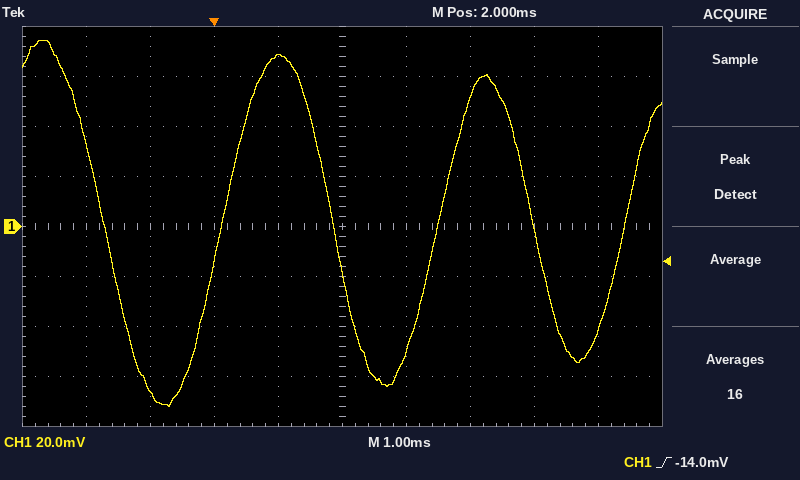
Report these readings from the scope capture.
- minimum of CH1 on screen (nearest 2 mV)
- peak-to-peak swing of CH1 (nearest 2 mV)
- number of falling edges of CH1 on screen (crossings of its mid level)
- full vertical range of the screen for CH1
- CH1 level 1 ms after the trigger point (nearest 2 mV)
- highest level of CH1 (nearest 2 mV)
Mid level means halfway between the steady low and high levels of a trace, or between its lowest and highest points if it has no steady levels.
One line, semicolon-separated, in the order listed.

-72 mV; 146 mV; 3; 160 mV; 68 mV; 74 mV
